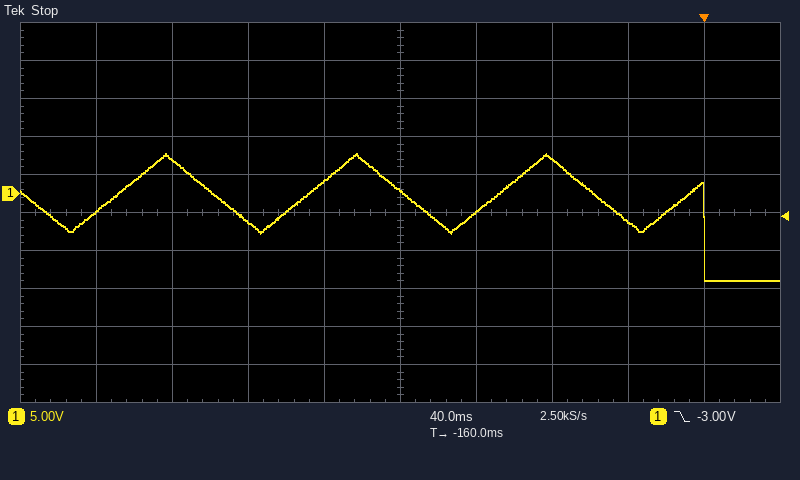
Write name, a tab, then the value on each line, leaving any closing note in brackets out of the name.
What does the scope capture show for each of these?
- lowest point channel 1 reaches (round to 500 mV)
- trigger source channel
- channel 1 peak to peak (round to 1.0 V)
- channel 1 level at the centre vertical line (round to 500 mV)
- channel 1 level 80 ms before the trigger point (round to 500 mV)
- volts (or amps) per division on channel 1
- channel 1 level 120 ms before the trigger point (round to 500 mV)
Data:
lowest point channel 1 reaches	-11.5 V
trigger source channel	channel 1
channel 1 peak to peak	17.0 V
channel 1 level at the centre vertical line	500 mV
channel 1 level 80 ms before the trigger point	4.5 V
volts (or amps) per division on channel 1	5 V
channel 1 level 120 ms before the trigger point	-2.5 V
